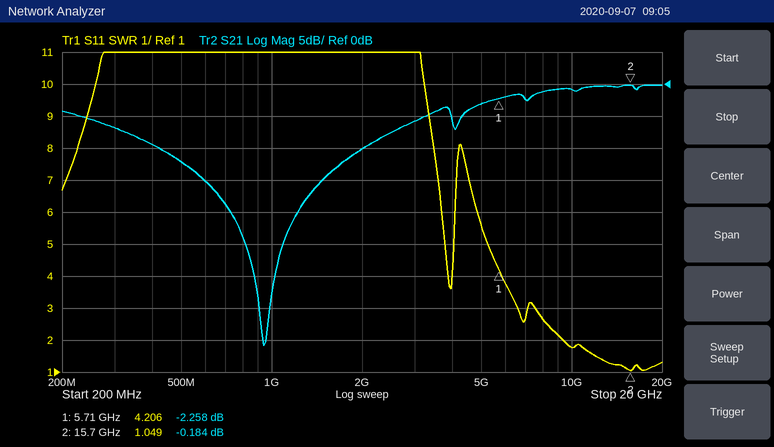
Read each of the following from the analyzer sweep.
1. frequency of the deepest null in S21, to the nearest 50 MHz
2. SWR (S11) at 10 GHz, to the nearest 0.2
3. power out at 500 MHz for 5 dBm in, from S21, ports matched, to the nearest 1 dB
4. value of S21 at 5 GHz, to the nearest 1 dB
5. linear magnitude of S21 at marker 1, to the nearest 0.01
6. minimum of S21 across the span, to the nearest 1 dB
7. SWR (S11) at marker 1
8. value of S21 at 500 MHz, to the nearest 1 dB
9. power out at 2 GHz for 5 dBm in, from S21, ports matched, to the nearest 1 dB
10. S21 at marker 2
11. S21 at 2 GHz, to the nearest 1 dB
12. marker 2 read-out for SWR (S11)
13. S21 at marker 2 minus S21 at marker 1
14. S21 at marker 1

950 MHz
1.8
-7 dBm
-3 dB
0.77
-41 dB
4.206
-12 dB
-5 dBm
-0.184 dB
-10 dB
1.049
2.074 dB
-2.258 dB
